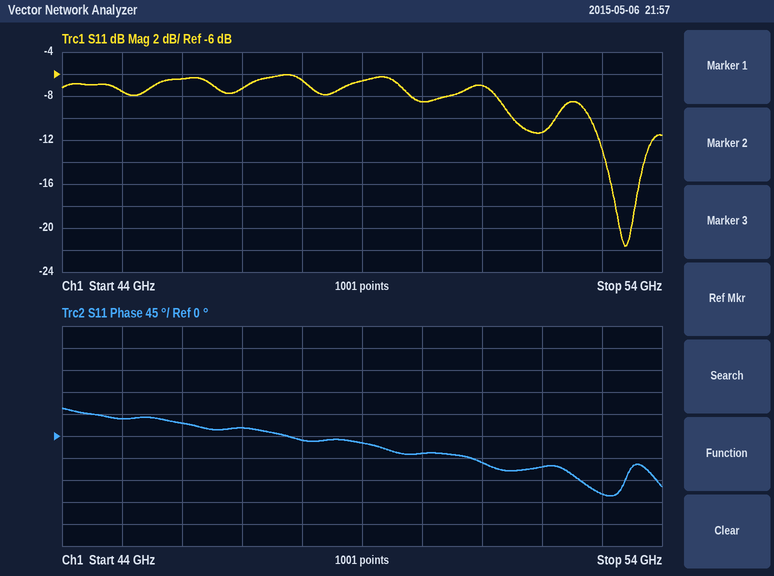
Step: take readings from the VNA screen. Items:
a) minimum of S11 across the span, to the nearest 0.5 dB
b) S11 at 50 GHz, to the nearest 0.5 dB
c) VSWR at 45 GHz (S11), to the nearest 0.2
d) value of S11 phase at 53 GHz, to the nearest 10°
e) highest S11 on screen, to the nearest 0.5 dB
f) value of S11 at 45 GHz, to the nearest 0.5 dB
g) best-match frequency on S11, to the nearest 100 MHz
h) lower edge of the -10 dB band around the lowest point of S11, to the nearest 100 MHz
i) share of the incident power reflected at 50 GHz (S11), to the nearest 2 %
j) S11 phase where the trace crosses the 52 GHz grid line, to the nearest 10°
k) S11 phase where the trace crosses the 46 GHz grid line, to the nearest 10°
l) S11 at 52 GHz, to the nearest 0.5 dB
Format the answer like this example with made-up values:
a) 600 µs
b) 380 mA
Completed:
a) -21.5 dB
b) -8.5 dB
c) 2.4
d) -120°
e) -6.0 dB
f) -7.5 dB
g) 53.4 GHz
h) 52.8 GHz
i) 14 %
j) -60°
k) 30°
l) -11.5 dB
